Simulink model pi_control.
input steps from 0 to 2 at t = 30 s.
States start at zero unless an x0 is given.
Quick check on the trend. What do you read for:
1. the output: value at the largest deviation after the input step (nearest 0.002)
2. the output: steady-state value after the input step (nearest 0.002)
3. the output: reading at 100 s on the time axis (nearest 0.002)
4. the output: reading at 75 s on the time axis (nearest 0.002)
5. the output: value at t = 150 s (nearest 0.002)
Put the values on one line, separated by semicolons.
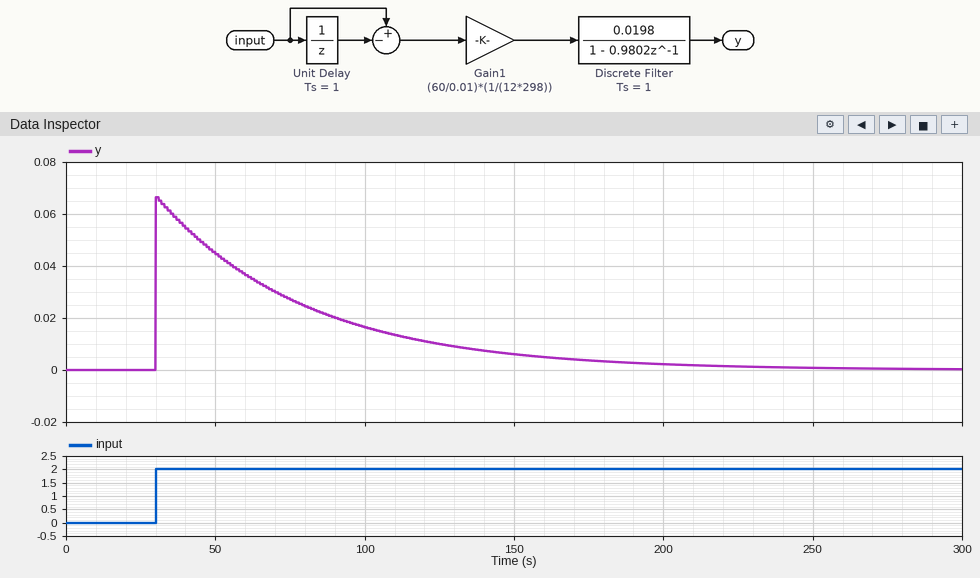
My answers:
0.066; 0.000; 0.016; 0.028; 0.006
